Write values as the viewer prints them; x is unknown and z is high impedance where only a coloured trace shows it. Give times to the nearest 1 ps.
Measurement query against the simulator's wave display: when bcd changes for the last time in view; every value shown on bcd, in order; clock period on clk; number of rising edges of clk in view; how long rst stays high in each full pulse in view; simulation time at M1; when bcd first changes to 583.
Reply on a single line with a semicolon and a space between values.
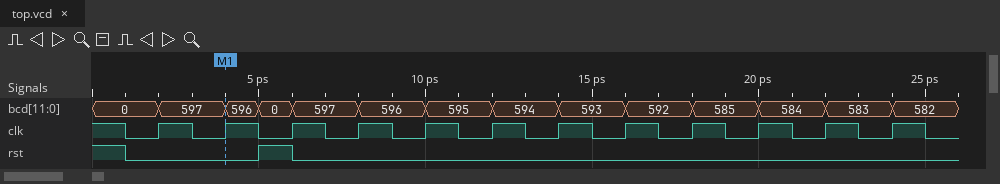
24 ps; 0, 597, 596, 0, 597, 596, 595, 594, 593, 592, 585, 584, 583, 582; 2 ps; 12; 1 ps; 4 ps; 22 ps
